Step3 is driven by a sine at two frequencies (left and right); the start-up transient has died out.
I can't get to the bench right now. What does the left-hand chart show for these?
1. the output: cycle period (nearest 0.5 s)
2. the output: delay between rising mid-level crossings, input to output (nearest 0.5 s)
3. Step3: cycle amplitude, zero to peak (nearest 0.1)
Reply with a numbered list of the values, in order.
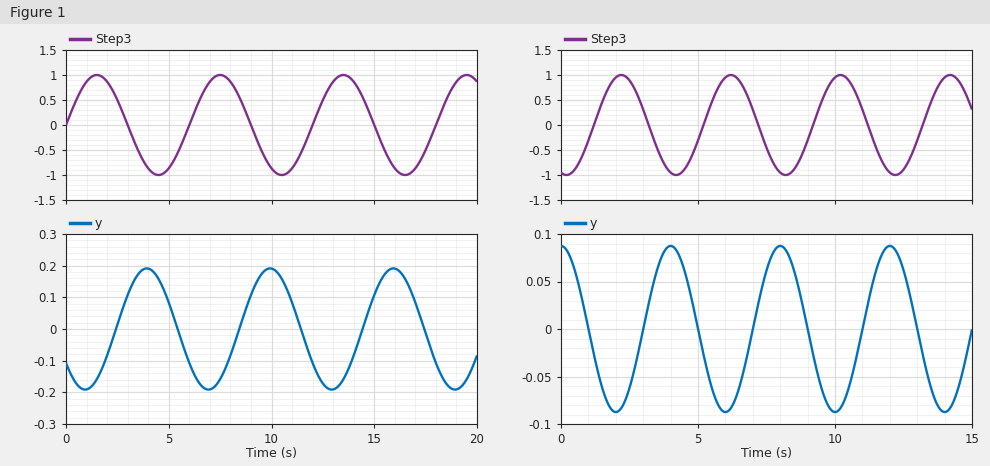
1. 6.0 s
2. 2.5 s
3. 1.0
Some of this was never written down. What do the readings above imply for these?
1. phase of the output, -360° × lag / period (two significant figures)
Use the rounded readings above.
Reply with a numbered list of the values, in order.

1. -150°
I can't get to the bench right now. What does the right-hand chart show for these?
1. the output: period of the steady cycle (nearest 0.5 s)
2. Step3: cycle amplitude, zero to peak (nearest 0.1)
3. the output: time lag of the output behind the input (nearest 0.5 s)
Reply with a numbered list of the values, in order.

1. 4.0 s
2. 1.0
3. 2.0 s
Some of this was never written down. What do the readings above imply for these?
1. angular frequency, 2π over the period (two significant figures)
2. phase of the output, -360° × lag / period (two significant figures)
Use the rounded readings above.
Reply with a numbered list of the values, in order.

1. 1.6 rad/s
2. -180°
